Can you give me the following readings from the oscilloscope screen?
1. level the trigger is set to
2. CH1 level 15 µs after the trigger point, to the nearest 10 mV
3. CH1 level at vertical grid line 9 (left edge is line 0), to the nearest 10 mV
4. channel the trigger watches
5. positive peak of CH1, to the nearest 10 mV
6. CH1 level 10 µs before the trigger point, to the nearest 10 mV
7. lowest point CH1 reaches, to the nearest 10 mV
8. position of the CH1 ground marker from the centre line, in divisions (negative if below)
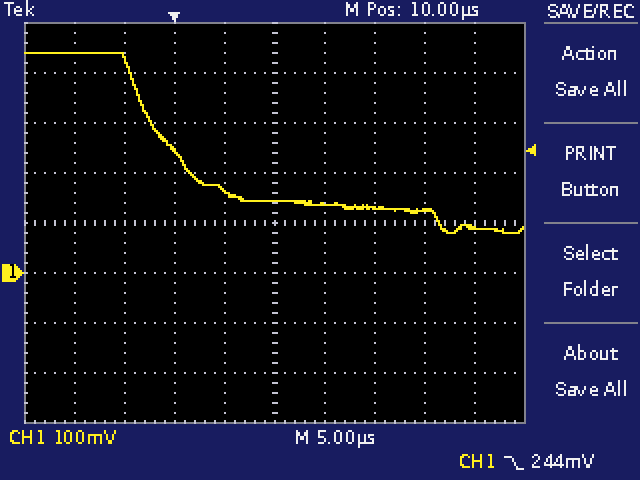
244 mV
140 mV
90 mV
CH1
440 mV
440 mV
80 mV
-1.0 div
